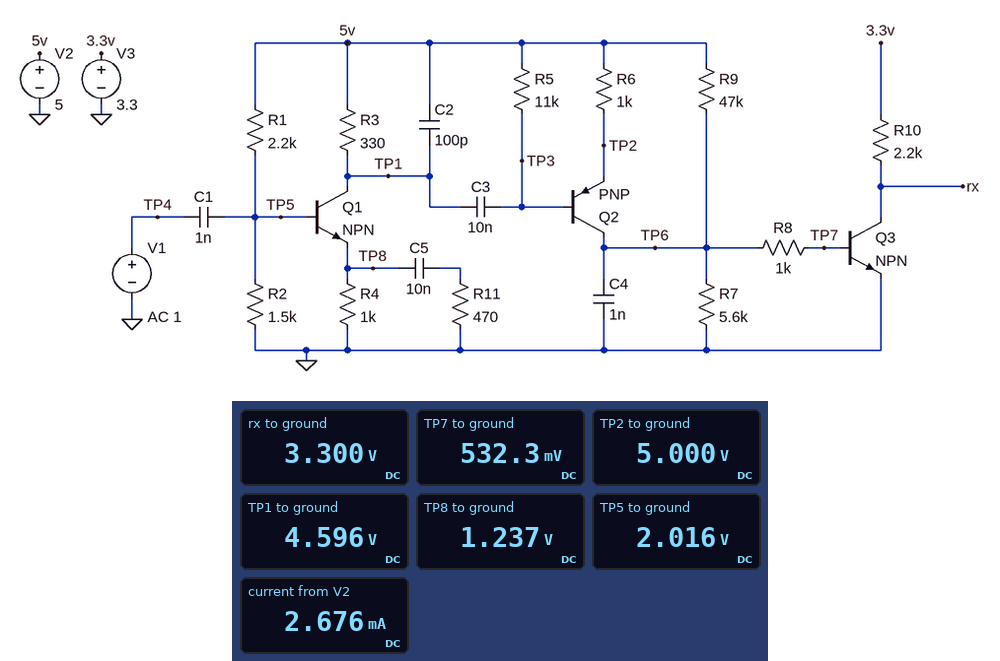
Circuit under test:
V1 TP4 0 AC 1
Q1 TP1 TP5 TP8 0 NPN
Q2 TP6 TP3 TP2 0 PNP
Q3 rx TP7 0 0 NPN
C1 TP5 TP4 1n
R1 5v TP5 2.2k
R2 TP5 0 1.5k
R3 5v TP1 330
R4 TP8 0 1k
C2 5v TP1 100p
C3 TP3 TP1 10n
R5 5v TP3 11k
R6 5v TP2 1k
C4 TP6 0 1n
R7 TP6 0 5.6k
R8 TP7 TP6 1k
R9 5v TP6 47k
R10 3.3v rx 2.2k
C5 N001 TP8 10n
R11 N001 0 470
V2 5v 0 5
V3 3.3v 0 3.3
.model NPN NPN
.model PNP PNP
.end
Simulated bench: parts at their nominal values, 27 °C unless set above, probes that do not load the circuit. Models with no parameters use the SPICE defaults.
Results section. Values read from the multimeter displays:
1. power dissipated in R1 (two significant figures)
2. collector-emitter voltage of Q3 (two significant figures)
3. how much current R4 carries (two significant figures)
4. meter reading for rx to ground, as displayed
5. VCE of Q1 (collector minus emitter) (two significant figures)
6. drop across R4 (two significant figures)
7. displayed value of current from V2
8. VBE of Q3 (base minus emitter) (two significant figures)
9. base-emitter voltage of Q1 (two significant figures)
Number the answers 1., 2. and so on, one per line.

1. 4.0 mW
2. 3.3 V
3. 1.2 mA
4. 3.300 V
5. 3.4 V
6. 1.2 V
7. 2.676 mA
8. 530 mV
9. 780 mV
